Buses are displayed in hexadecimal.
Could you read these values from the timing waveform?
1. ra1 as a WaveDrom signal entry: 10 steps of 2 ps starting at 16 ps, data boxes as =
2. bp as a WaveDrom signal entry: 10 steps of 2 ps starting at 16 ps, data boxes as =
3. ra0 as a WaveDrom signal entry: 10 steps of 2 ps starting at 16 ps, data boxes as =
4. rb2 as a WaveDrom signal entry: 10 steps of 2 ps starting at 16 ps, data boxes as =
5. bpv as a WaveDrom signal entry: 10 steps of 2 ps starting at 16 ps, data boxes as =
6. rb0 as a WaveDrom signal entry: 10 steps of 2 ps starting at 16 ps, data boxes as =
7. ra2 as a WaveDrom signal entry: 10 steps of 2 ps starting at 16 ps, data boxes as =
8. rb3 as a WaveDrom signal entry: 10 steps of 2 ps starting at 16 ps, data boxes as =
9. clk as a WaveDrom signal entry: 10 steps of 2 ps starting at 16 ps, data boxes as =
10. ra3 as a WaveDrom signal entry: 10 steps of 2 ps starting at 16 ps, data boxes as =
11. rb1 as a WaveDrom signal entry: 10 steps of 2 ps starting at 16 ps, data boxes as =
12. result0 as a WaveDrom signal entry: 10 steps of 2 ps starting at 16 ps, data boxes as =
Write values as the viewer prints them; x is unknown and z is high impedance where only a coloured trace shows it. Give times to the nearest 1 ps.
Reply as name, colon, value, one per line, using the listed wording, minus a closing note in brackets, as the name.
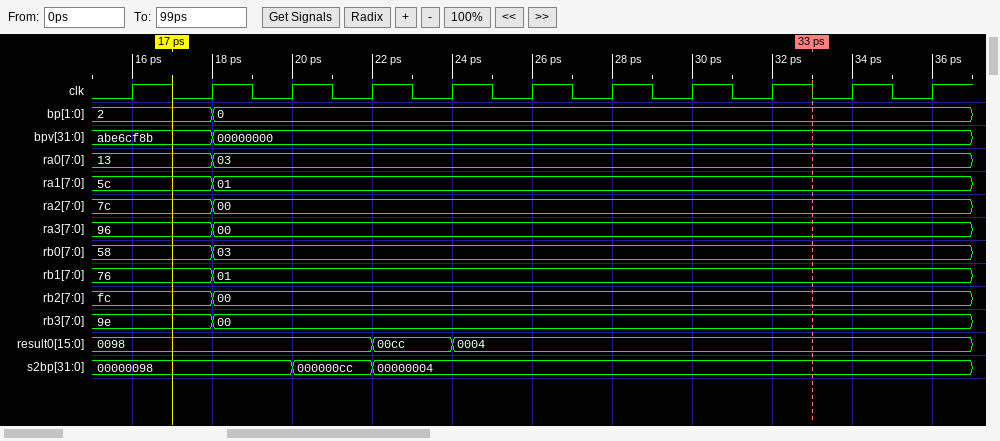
ra1 as a WaveDrom signal entry: 10 steps of 2 ps starting at 16 ps, data boxes as =: {name: 'ra1', wave: '==........', data: '5c 01'}
bp as a WaveDrom signal entry: 10 steps of 2 ps starting at 16 ps, data boxes as =: {name: 'bp', wave: '==........', data: '2 0'}
ra0 as a WaveDrom signal entry: 10 steps of 2 ps starting at 16 ps, data boxes as =: {name: 'ra0', wave: '==........', data: '13 03'}
rb2 as a WaveDrom signal entry: 10 steps of 2 ps starting at 16 ps, data boxes as =: {name: 'rb2', wave: '==........', data: 'fc 00'}
bpv as a WaveDrom signal entry: 10 steps of 2 ps starting at 16 ps, data boxes as =: {name: 'bpv', wave: '==........', data: 'abe6cf8b 00000000'}
rb0 as a WaveDrom signal entry: 10 steps of 2 ps starting at 16 ps, data boxes as =: {name: 'rb0', wave: '==........', data: '58 03'}
ra2 as a WaveDrom signal entry: 10 steps of 2 ps starting at 16 ps, data boxes as =: {name: 'ra2', wave: '==........', data: '7c 00'}
rb3 as a WaveDrom signal entry: 10 steps of 2 ps starting at 16 ps, data boxes as =: {name: 'rb3', wave: '==........', data: '9e 00'}
clk as a WaveDrom signal entry: 10 steps of 2 ps starting at 16 ps, data boxes as =: {name: 'clk', wave: 'p.........'}
ra3 as a WaveDrom signal entry: 10 steps of 2 ps starting at 16 ps, data boxes as =: {name: 'ra3', wave: '==........', data: '96 00'}
rb1 as a WaveDrom signal entry: 10 steps of 2 ps starting at 16 ps, data boxes as =: {name: 'rb1', wave: '==........', data: '76 01'}
result0 as a WaveDrom signal entry: 10 steps of 2 ps starting at 16 ps, data boxes as =: {name: 'result0', wave: '=..==.....', data: '0098 00cc 0004'}
